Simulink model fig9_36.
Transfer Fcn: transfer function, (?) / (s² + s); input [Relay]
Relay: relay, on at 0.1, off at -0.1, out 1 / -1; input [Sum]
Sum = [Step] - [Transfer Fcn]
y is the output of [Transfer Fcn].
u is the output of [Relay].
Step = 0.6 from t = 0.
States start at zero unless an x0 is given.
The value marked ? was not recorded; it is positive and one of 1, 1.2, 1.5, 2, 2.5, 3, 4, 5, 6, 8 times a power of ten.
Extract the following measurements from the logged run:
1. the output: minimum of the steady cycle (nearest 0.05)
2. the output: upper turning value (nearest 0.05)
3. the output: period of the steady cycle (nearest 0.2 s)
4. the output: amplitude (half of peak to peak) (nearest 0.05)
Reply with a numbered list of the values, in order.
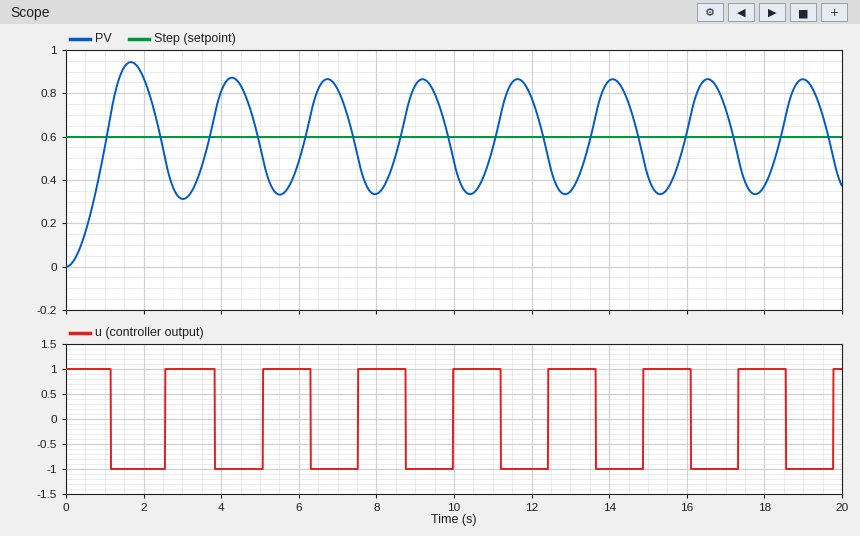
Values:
1. 0.35
2. 0.85
3. 2.4 s
4. 0.25
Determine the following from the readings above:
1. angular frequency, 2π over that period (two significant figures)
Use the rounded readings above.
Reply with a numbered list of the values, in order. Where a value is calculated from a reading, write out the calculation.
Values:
1. 2π / 2.4 = 2.6 rad/s
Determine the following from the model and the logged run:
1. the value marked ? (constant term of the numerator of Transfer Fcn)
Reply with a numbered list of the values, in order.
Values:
1. 1.5
